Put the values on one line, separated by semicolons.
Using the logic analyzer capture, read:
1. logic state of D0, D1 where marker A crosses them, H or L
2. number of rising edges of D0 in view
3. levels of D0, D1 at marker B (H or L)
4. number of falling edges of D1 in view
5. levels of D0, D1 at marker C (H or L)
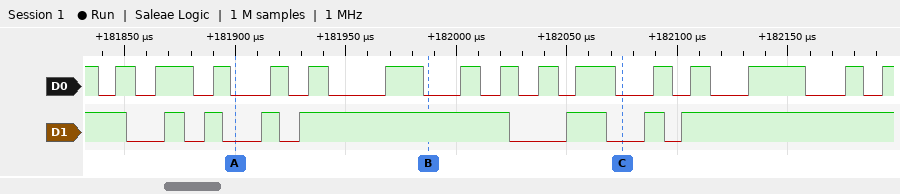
D0=L, D1=L; 15; D0=L, D1=H; 7; D0=L, D1=L
